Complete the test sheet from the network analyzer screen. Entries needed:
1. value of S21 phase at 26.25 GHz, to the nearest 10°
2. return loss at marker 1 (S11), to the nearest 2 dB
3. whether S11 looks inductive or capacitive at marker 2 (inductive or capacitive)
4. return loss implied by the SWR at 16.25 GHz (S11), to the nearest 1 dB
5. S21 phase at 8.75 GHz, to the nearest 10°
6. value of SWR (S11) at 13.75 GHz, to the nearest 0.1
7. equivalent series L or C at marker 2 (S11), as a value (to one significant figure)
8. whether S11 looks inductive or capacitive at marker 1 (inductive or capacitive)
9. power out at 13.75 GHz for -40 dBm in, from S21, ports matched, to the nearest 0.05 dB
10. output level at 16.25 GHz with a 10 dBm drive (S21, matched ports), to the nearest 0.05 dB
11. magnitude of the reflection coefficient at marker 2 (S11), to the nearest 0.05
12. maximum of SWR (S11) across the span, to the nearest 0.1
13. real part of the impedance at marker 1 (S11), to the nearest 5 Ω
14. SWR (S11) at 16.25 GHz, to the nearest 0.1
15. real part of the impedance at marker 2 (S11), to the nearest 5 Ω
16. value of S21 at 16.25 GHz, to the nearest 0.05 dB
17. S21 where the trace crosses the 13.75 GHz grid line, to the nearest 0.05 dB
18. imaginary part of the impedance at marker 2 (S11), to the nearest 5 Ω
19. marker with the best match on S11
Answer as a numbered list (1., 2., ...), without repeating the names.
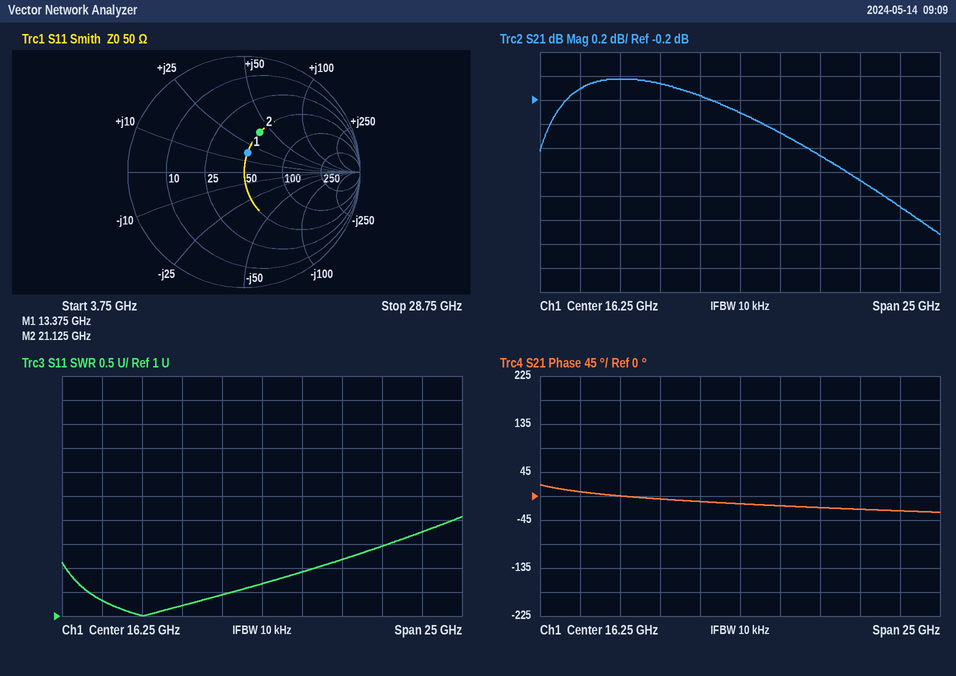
1. -30°
2. 16 dB
3. inductive
4. 12 dB
5. 0°
6. 1.4
7. 300 pH
8. inductive
9. -40.15 dBm
10. 9.70 dBm
11. 0.35
12. 3.1
13. 50 Ω
14. 1.7
15. 50 Ω
16. -0.30 dB
17. -0.15 dB
18. +40 Ω
19. marker 1
